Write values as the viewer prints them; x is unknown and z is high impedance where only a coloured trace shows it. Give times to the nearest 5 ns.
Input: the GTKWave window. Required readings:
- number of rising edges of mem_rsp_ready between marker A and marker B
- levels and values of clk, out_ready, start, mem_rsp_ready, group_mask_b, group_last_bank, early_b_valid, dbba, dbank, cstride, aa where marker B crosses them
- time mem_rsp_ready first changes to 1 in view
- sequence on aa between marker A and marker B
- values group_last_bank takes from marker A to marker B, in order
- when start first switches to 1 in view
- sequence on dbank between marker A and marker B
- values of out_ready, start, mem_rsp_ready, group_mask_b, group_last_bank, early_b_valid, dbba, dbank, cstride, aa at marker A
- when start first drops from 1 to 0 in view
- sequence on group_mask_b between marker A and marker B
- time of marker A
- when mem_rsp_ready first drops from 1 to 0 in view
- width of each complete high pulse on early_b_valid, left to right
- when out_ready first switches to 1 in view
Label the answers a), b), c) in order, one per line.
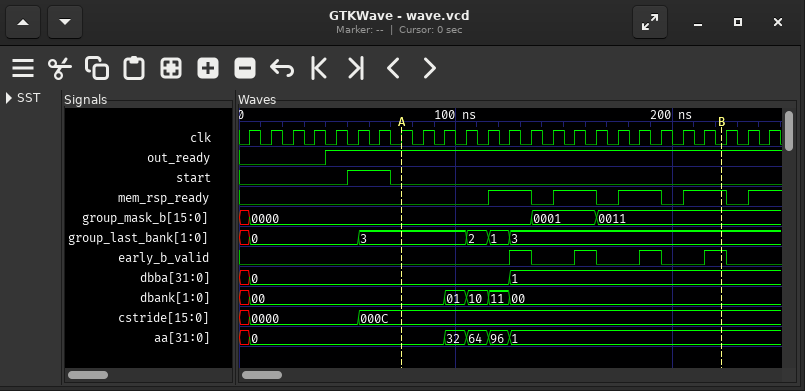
a) 4
b) clk=0, out_ready=1, start=0, mem_rsp_ready=1, group_mask_b=0011, group_last_bank=3, early_b_valid=1, dbba=1, dbank=00, cstride=000C, aa=1
c) 115 ns
d) 0, 32, 64, 96, 1
e) 3, 2, 1, 3
f) 50 ns
g) 00, 01, 10, 11, 00
h) out_ready=1, start=0, mem_rsp_ready=0, group_mask_b=0000, group_last_bank=3, early_b_valid=0, dbba=0, dbank=00, cstride=000C, aa=0
i) 70 ns
j) 0000, 0001, 0011
k) 75 ns
l) 135 ns
m) 10 ns, 10 ns, 10 ns, 10 ns
n) 40 ns
